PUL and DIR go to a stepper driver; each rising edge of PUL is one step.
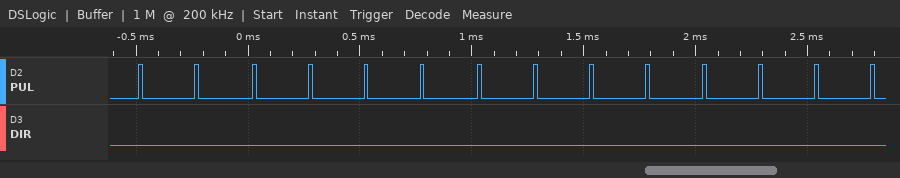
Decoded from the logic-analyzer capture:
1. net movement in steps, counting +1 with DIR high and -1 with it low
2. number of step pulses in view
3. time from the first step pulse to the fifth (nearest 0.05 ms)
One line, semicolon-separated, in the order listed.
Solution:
-14; 14; 1.00 ms
